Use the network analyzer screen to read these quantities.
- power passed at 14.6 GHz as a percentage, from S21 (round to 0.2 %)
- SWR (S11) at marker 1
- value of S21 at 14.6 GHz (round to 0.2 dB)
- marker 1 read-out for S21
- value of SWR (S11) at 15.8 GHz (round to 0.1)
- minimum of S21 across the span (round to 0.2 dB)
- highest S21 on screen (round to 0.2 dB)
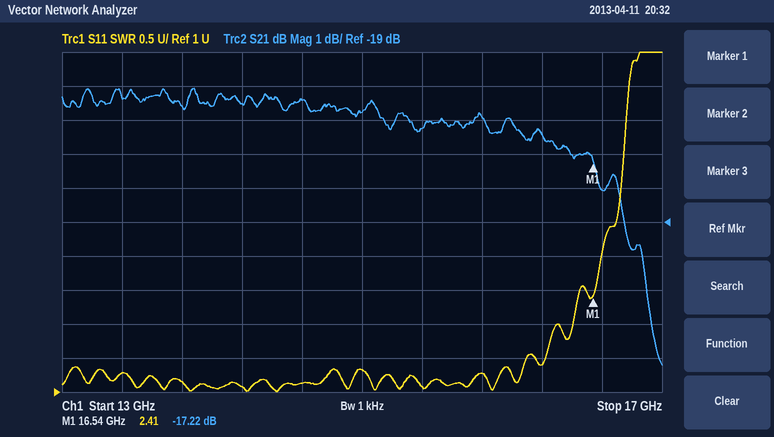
2.8 %
2.41
-15.4 dB
-17.22 dB
1.3
-23.2 dB
-15.0 dB
